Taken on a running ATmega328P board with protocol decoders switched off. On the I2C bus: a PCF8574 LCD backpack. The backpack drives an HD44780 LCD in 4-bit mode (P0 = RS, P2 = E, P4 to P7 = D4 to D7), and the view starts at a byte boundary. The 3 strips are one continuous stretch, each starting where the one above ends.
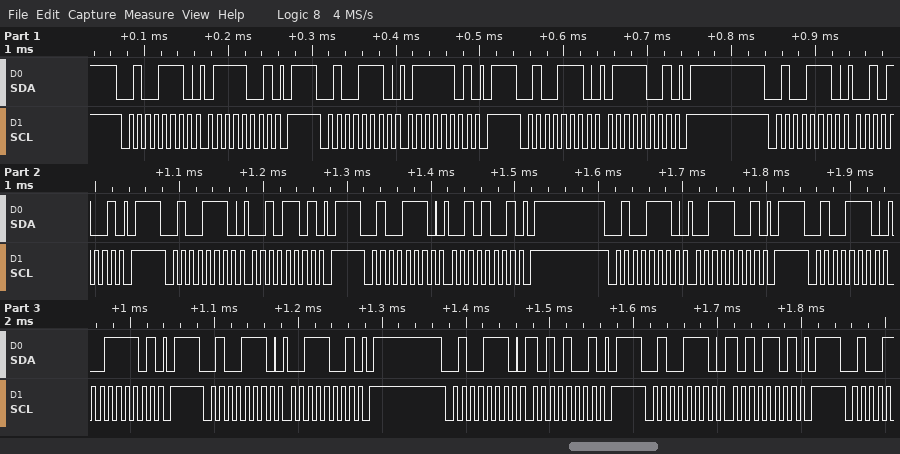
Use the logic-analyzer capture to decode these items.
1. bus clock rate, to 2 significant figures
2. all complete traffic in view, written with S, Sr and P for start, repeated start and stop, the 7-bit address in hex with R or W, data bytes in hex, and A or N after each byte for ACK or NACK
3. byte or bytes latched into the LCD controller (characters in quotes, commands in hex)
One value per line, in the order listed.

100 kHz
S 27W A 79 A P S 27W A 7D A P S 27W A 79 A P S 27W A 29 A P S 27W A 2D A P S 27W A 29 A P S 27W A 39 A P S 27W A 3D A P S 27W A 39 A P S 27W A A9 A P S 27W A AD A P
'r'
